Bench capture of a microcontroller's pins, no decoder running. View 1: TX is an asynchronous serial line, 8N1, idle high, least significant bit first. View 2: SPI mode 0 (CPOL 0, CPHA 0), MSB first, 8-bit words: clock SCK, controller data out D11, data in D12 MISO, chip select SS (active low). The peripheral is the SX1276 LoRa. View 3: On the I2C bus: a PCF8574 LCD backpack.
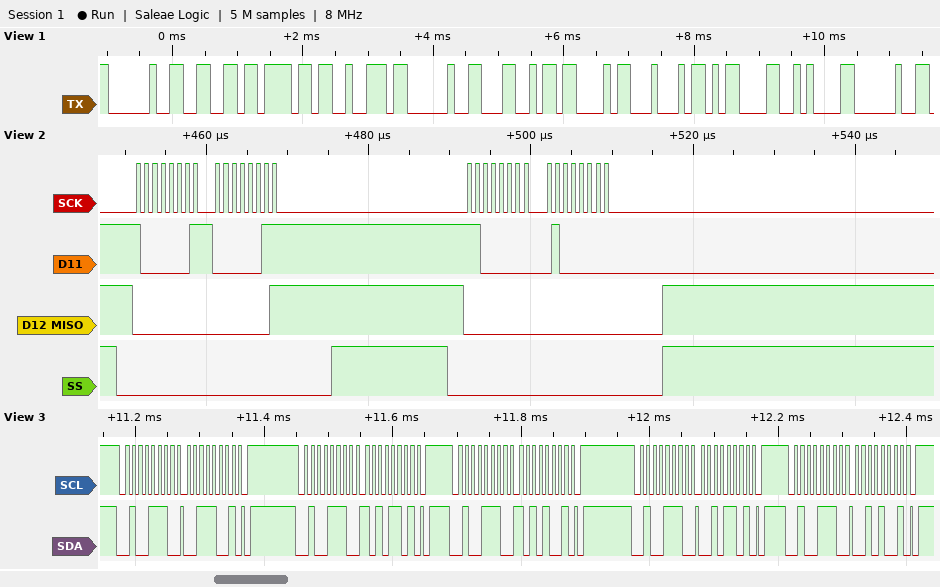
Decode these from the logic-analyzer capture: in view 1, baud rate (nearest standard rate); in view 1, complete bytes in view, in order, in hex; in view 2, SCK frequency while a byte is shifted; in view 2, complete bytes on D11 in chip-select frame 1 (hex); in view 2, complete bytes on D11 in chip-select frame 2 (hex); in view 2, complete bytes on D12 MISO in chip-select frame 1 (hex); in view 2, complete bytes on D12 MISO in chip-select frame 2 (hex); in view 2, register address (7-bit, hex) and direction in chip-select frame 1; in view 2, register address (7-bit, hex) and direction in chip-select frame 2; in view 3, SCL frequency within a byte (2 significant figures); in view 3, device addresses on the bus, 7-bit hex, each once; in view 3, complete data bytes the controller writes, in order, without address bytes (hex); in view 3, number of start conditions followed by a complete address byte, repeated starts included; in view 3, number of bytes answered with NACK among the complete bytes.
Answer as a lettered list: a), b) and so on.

a) 9600 baud
b) 0x20 0x66 0x6F 0x72 0x20 0x4C 0x43 0x44 0x0D 0x0A 0x20
c) 1 MHz
d) 81 03
e) C0 40
f) 00 01
g) 00 00
h) 0x01 write
i) 0x40 write
j) 100 kHz
k) 0x27
l) 39 AD A9 2D 29
m) 5
n) 0
